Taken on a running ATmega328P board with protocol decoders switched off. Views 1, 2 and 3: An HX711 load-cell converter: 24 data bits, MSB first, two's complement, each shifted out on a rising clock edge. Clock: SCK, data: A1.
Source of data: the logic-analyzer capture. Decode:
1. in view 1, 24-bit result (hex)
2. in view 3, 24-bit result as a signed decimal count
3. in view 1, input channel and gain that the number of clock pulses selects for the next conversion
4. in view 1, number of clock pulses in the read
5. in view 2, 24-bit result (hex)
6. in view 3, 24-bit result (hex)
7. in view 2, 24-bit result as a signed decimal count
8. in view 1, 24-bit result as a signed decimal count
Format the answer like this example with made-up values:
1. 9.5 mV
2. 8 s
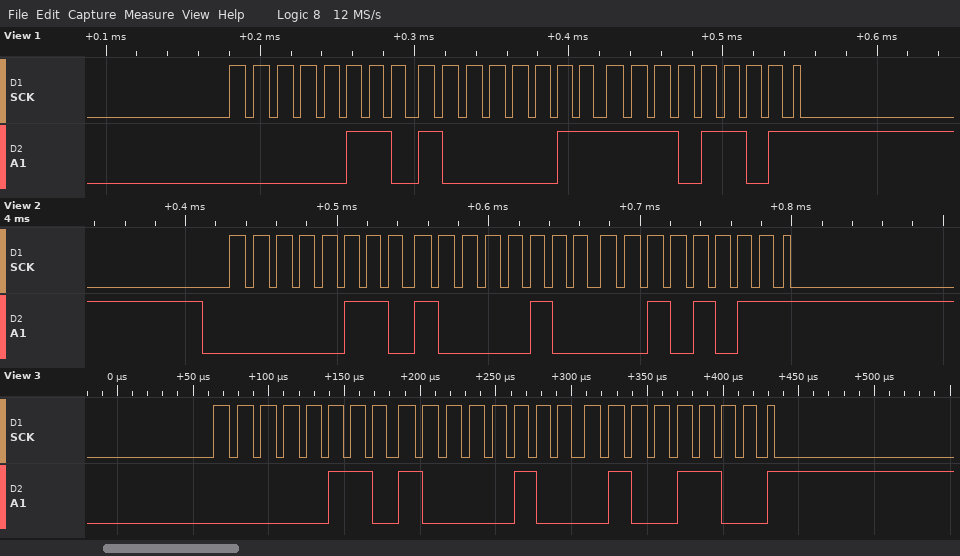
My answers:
1. 0x0683ED
2. 427084
3. channel A, gain 128
4. 25
5. 0x06842B
6. 0x06844C
7. 427051
8. 426989
